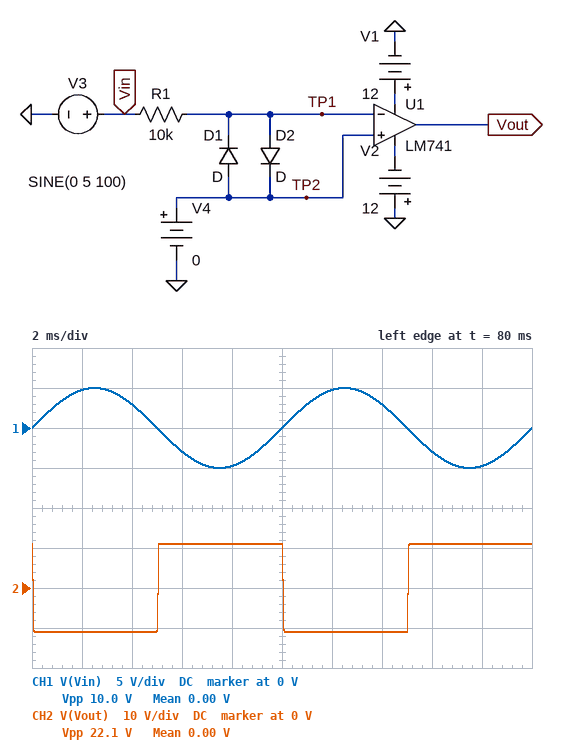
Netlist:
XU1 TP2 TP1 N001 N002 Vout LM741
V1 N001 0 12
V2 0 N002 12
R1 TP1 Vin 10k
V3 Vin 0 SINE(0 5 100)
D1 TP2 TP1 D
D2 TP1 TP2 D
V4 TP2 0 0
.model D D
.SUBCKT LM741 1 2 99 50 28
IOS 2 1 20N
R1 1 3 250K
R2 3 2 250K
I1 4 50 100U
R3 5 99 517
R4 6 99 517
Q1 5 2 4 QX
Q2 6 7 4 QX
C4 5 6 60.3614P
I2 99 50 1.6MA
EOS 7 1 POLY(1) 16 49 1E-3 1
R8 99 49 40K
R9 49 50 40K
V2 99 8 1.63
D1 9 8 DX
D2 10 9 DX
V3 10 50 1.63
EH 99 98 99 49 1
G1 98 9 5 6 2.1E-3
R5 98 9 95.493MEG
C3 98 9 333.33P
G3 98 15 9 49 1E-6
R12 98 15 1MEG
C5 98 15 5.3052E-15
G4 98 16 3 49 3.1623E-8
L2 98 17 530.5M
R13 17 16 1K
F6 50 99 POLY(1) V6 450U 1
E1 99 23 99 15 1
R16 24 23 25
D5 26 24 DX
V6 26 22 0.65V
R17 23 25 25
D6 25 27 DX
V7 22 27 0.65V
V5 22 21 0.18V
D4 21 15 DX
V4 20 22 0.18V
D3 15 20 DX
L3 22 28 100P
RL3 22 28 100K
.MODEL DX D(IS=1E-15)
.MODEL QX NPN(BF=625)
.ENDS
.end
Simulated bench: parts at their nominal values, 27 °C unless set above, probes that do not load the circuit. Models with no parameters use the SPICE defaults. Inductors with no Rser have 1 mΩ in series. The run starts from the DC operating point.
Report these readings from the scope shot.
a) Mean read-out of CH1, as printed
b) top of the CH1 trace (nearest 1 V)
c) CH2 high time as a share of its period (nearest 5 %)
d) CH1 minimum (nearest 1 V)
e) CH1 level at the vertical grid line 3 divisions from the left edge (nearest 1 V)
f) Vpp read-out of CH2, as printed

0.00 V
5 V
50 %
-5 V
-3 V
22.1 V
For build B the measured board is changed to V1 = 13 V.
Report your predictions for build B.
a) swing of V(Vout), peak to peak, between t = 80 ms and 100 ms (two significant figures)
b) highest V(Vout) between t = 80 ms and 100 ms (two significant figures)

23 V
12 V
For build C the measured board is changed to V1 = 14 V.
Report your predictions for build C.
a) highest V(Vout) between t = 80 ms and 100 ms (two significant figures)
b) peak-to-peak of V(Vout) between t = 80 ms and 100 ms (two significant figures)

13 V
24 V
